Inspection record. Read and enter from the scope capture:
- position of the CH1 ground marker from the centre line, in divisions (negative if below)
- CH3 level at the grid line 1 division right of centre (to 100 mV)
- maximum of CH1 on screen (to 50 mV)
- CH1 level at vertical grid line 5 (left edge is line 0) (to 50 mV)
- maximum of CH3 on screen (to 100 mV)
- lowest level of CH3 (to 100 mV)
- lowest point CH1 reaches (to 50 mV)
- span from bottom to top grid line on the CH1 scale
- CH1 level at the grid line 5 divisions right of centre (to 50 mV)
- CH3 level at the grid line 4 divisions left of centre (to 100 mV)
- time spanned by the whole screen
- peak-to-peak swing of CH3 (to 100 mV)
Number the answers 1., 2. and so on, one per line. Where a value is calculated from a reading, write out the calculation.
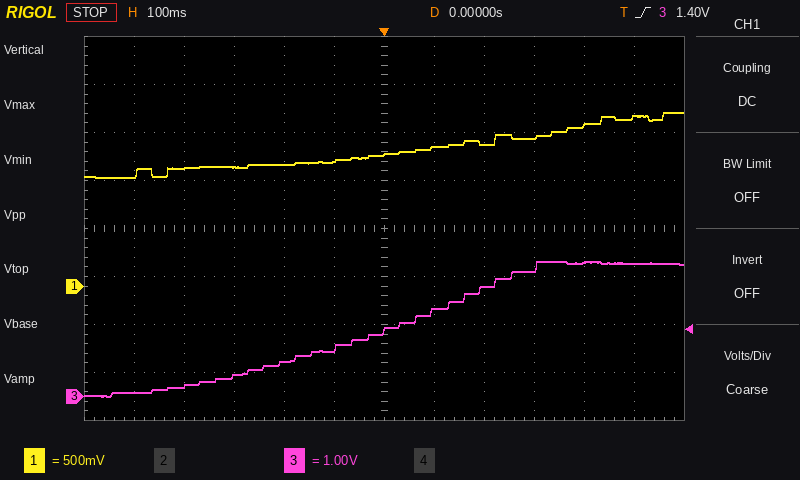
1. -1.2 div
2. 1.8 V
3. 1.80 V
4. 1.30 V
5. 2.8 V
6. 0.0 V
7. 1.15 V
8. 4 V
9. 1.75 V
10. 200 mV
11. 1.2 s
12. 2.8 V − (0.0 V) = 2.8 V
